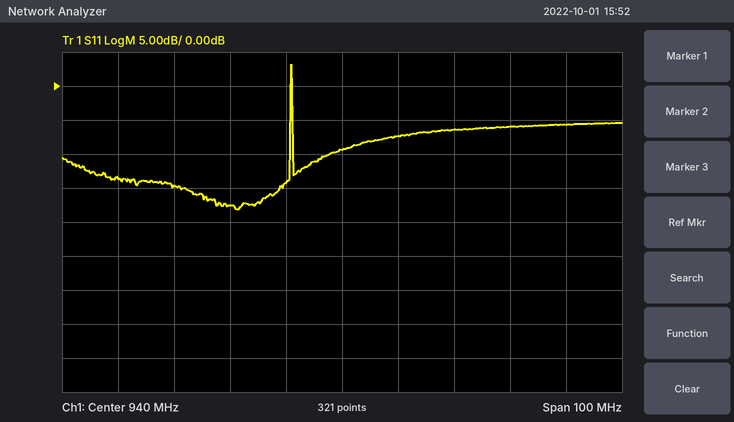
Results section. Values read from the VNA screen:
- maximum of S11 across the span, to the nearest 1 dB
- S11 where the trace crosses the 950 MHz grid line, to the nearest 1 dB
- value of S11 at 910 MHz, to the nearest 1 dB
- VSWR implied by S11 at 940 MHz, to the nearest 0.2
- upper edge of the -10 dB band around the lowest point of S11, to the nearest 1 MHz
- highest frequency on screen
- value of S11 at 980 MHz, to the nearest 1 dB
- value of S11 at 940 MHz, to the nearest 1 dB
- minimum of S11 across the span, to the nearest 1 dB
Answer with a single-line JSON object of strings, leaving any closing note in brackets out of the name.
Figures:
{"maximum of S11 across the span, to the nearest 1 dB": "3 dB", "S11 where the trace crosses the 950 MHz grid line, to the nearest 1 dB": "-7 dB", "value of S11 at 910 MHz, to the nearest 1 dB": "-15 dB", "VSWR implied by S11 at 940 MHz, to the nearest 0.2": "2.0", "upper edge of the -10 dB band around the lowest point of S11, to the nearest 1 MHz": "931 MHz", "highest frequency on screen": "990 MHz", "value of S11 at 980 MHz, to the nearest 1 dB": "-6 dB", "value of S11 at 940 MHz, to the nearest 1 dB": "-9 dB", "minimum of S11 across the span, to the nearest 1 dB": "-18 dB"}
